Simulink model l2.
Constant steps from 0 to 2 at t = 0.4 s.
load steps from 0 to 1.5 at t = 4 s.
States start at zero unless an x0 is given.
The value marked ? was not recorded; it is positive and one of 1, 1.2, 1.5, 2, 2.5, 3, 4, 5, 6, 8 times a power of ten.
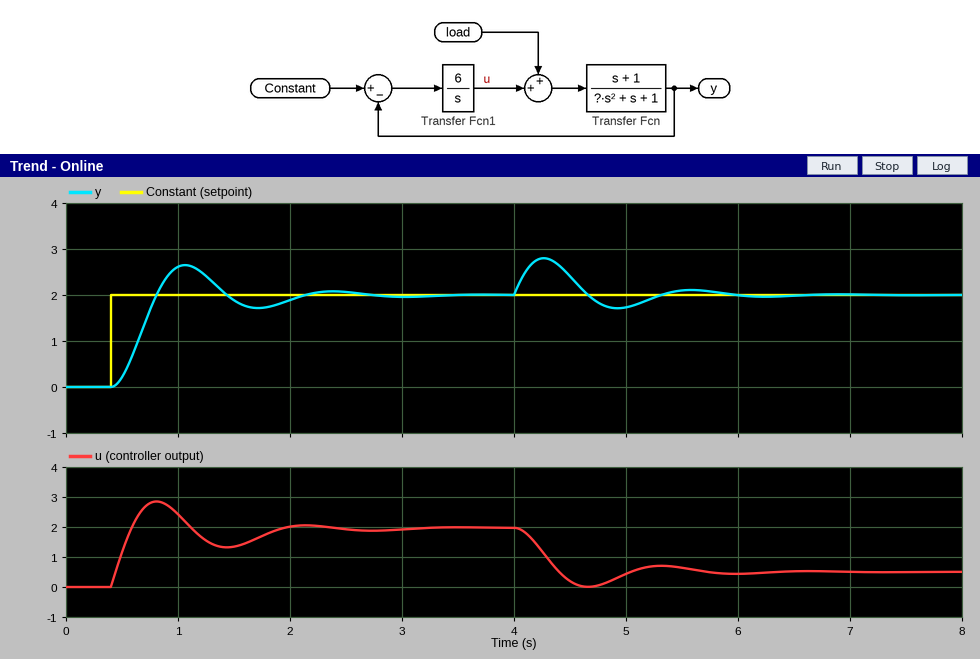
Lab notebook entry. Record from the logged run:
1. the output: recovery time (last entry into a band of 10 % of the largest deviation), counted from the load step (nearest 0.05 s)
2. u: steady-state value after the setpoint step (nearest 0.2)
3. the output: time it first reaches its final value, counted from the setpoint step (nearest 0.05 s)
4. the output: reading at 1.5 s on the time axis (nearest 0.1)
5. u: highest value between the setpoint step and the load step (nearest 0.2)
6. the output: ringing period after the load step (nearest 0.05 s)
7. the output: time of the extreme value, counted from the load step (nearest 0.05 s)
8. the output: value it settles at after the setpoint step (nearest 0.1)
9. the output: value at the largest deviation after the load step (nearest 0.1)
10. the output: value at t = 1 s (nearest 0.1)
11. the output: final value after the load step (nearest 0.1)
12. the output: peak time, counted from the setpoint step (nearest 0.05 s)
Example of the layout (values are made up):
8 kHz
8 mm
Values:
1.75 s
2.0
0.40 s
1.9
2.8
1.30 s
0.25 s
2.0
2.8
2.6
2.0
0.65 s
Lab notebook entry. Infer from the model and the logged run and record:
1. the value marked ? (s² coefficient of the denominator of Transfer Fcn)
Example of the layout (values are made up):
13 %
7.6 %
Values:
0.25
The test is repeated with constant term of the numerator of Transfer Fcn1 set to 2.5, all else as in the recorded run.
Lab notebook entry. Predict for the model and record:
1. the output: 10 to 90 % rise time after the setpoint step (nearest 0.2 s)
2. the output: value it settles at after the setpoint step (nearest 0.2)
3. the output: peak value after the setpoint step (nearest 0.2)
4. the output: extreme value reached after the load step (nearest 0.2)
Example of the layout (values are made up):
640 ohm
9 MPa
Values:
0.6 s
2.0
2.2
3.0
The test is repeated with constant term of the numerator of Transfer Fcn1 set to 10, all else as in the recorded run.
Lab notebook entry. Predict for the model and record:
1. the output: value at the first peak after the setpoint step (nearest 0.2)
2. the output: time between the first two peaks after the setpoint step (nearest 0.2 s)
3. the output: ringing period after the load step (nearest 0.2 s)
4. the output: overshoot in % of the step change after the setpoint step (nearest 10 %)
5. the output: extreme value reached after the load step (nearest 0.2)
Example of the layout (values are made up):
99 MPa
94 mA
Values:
2.8
1.0 s
1.0 s
40 %
2.6
